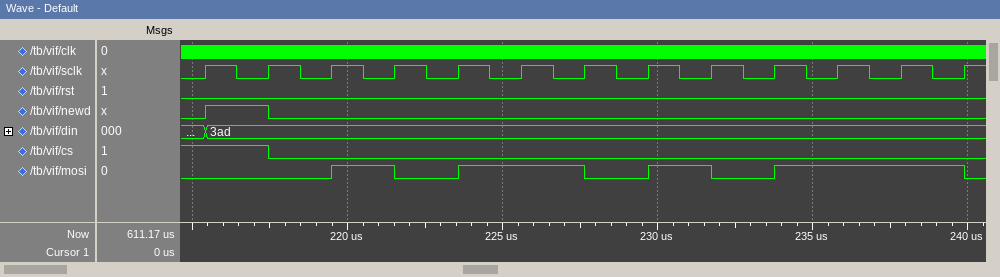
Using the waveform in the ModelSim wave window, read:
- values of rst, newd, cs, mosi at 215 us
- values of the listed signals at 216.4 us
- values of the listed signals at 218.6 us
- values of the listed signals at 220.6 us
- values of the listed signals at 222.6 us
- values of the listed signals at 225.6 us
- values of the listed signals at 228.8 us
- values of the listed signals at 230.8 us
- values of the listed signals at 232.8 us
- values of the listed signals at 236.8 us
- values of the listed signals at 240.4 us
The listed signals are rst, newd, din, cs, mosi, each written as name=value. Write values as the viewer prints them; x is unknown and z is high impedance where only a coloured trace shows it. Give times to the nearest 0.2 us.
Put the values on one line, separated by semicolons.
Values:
rst=0, newd=0, cs=1, mosi=0; rst=0, newd=1, din=3ad, cs=1, mosi=0; rst=0, newd=0, din=3ad, cs=0, mosi=0; rst=0, newd=0, din=3ad, cs=0, mosi=1; rst=0, newd=0, din=3ad, cs=0, mosi=0; rst=0, newd=0, din=3ad, cs=0, mosi=1; rst=0, newd=0, din=3ad, cs=0, mosi=0; rst=0, newd=0, din=3ad, cs=0, mosi=1; rst=0, newd=0, din=3ad, cs=0, mosi=0; rst=0, newd=0, din=3ad, cs=0, mosi=1; rst=0, newd=0, din=3ad, cs=0, mosi=0
